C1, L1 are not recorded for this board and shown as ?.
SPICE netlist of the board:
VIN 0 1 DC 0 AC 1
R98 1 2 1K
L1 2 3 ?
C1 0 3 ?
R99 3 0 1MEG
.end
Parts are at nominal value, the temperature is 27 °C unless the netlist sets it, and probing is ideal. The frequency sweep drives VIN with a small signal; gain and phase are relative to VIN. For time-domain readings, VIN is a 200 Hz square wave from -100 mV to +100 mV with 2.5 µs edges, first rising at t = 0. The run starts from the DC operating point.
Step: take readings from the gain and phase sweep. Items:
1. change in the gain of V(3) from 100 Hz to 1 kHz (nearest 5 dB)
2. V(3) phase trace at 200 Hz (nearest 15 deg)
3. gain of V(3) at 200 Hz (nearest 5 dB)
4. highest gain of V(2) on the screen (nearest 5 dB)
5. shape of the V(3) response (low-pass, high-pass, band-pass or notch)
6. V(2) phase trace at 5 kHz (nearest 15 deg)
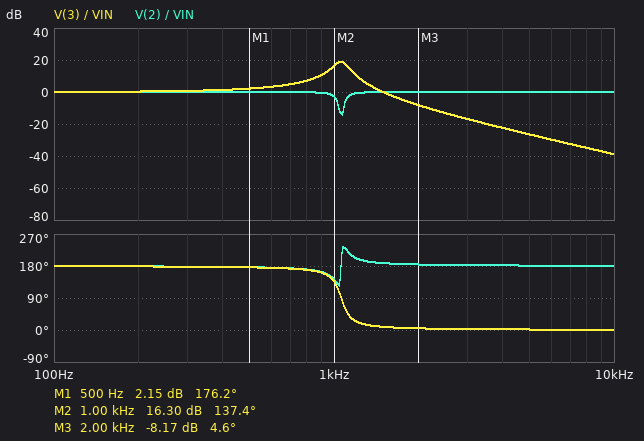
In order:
15 dB
180 deg
0 dB
0 dB
band-pass
180 deg
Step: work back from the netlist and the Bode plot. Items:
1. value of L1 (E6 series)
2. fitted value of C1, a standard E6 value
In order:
1.5 H
15 nF
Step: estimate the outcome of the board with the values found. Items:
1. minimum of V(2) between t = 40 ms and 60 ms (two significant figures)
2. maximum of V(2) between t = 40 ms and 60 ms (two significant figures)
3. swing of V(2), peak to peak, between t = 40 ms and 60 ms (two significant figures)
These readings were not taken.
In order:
-120 mV
120 mV
240 mV
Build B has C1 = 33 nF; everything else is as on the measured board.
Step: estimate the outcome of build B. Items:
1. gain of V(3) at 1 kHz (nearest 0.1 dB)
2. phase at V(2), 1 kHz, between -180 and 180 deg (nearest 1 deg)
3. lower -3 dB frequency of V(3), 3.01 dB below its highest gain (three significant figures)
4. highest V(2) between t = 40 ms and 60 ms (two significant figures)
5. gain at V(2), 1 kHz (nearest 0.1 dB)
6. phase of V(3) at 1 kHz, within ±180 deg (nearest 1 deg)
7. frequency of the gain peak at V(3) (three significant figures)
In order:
0.2 dB
-168 deg
653 Hz
120 mV
-0.2 dB
13 deg
711 Hz
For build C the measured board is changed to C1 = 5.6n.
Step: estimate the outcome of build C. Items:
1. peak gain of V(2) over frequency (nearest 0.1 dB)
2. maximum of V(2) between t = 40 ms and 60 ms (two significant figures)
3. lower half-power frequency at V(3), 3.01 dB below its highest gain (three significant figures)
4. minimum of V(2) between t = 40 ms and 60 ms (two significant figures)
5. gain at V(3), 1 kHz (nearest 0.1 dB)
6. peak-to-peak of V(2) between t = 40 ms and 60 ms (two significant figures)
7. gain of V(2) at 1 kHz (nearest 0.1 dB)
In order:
0 dB
110 mV
1.67 kHz
-110 mV
3.5 dB
220 mV
0 dB
